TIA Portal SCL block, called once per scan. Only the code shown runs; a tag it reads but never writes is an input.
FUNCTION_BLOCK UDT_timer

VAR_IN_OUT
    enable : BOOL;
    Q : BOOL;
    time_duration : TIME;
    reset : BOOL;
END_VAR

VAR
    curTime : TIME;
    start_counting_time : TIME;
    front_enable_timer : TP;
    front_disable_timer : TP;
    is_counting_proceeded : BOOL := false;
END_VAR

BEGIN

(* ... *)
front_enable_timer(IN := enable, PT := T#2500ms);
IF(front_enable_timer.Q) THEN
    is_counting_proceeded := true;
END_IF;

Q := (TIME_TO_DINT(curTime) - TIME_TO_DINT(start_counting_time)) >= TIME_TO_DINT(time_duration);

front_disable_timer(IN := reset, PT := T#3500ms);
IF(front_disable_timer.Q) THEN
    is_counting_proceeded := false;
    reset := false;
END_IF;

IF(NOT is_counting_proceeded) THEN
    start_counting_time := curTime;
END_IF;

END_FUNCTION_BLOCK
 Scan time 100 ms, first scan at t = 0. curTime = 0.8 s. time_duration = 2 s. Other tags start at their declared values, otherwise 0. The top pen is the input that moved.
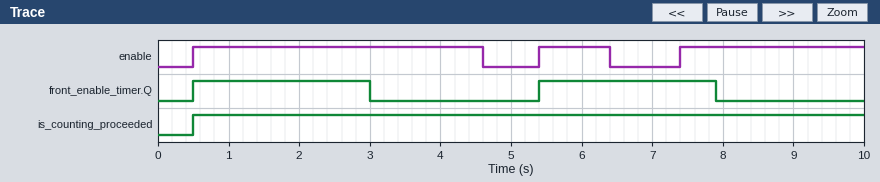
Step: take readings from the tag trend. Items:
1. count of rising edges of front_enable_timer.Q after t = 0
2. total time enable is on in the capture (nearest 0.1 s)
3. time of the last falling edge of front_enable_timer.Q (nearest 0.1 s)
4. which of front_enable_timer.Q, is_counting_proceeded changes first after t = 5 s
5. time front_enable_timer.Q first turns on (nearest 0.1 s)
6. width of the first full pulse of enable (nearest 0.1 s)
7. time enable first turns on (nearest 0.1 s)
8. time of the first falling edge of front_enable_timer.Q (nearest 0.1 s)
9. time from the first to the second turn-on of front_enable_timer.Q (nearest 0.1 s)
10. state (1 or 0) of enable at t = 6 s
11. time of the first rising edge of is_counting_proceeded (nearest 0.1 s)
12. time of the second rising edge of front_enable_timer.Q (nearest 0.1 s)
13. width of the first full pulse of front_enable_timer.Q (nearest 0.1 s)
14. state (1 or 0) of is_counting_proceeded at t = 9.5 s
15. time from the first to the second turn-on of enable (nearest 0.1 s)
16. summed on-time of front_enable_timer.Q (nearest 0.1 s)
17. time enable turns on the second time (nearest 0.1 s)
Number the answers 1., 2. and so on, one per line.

1. 2
2. 7.7 s
3. 7.9 s
4. front_enable_timer.Q
5. 0.5 s
6. 4.1 s
7. 0.5 s
8. 3.0 s
9. 4.9 s
10. 1
11. 0.5 s
12. 5.4 s
13. 2.5 s
14. 1
15. 4.9 s
16. 5.0 s
17. 5.4 s
